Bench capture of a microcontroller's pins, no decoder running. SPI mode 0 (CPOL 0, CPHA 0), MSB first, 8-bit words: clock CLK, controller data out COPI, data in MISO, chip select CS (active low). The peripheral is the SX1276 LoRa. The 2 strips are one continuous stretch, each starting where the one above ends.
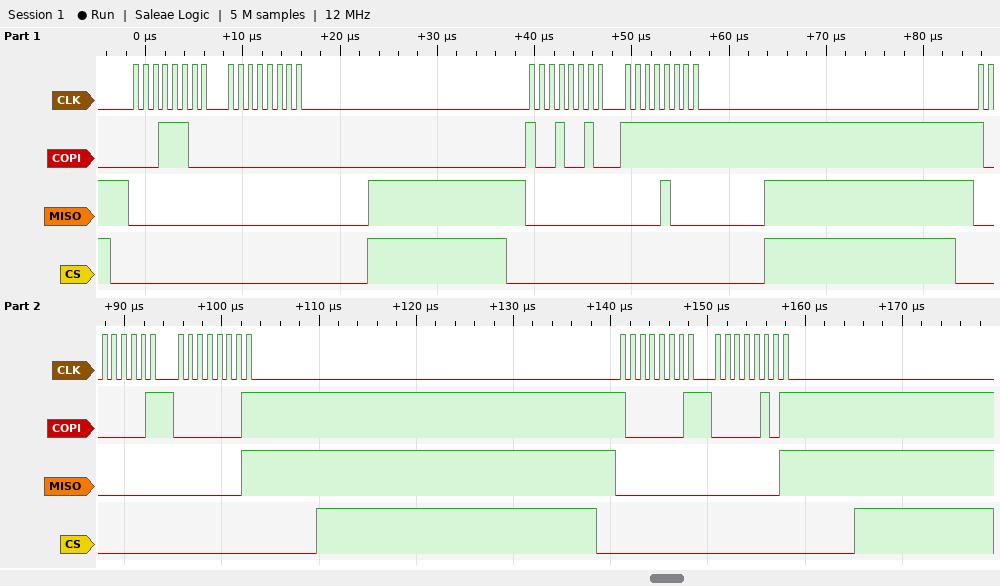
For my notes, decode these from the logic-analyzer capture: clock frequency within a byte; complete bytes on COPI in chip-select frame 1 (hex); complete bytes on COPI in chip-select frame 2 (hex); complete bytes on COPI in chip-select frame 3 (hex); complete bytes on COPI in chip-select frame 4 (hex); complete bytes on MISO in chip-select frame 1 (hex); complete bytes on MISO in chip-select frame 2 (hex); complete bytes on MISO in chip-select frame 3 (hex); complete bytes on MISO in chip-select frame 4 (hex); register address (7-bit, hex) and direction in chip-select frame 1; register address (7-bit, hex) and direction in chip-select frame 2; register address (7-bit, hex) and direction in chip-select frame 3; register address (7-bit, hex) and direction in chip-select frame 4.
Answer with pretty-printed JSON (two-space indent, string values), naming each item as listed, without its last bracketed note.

{
  "clock frequency within a byte": "1 MHz",
  "complete bytes on COPI in chip-select frame 1": "1C 00",
  "complete bytes on COPI in chip-select frame 2": "92 FF",
  "complete bytes on COPI in chip-select frame 3": "81 01",
  "complete bytes on COPI in chip-select frame 4": "81 05",
  "complete bytes on MISO in chip-select frame 1": "00 00",
  "complete bytes on MISO in chip-select frame 2": "00 08",
  "complete bytes on MISO in chip-select frame 3": "00 01",
  "complete bytes on MISO in chip-select frame 4": "00 01",
  "register address (7-bit, hex) and direction in chip-select frame 1": "0x1C read",
  "register address (7-bit, hex) and direction in chip-select frame 2": "0x12 write",
  "register address (7-bit, hex) and direction in chip-select frame 3": "0x01 write",
  "register address (7-bit, hex) and direction in chip-select frame 4": "0x01 write"
}
